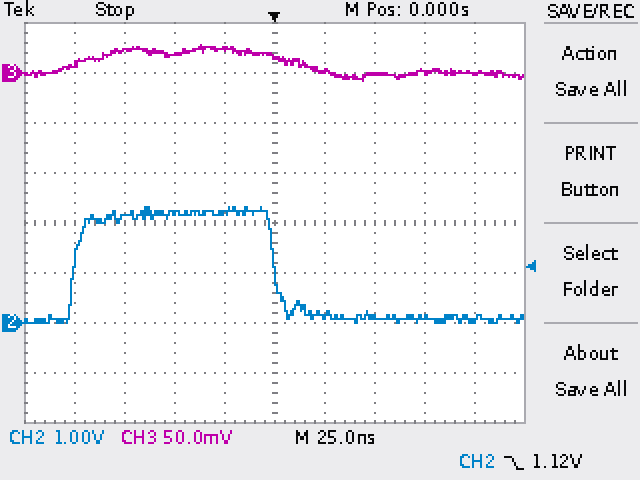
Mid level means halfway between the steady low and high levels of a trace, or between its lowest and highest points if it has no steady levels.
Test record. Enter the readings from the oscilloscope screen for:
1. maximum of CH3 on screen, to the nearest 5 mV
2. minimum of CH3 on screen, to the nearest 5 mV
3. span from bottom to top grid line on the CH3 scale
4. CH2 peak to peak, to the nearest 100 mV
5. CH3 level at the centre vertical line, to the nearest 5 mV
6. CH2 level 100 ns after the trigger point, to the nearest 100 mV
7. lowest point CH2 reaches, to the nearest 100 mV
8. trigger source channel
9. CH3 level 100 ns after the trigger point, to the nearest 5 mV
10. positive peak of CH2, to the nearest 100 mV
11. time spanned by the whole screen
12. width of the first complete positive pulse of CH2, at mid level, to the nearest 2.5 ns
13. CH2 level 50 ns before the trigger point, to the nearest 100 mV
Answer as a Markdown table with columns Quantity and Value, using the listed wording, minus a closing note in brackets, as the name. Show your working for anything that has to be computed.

| Quantity | Value |
|---|---|
| maximum of CH3 on screen, to the nearest 5 mV | 30 mV |
| minimum of CH3 on screen, to the nearest 5 mV | -10 mV |
| span from bottom to top grid line on the CH3 scale | 400 mV |
| CH2 peak to peak, to the nearest 100 mV | 2.3 V − (0.0 V) = 2.3 V |
| CH3 level at the centre vertical line, to the nearest 5 mV | 15 mV |
| CH2 level 100 ns after the trigger point, to the nearest 100 mV | 100 mV |
| lowest point CH2 reaches, to the nearest 100 mV | 0.0 V |
| trigger source channel | CH2 |
| CH3 level 100 ns after the trigger point, to the nearest 5 mV | 0 mV |
| positive peak of CH2, to the nearest 100 mV | 2.3 V |
| time spanned by the whole screen | 250 ns |
| width of the first complete positive pulse of CH2, at mid level, to the nearest 2.5 ns | 100.0 ns |
| CH2 level 50 ns before the trigger point, to the nearest 100 mV | 2.2 V |
